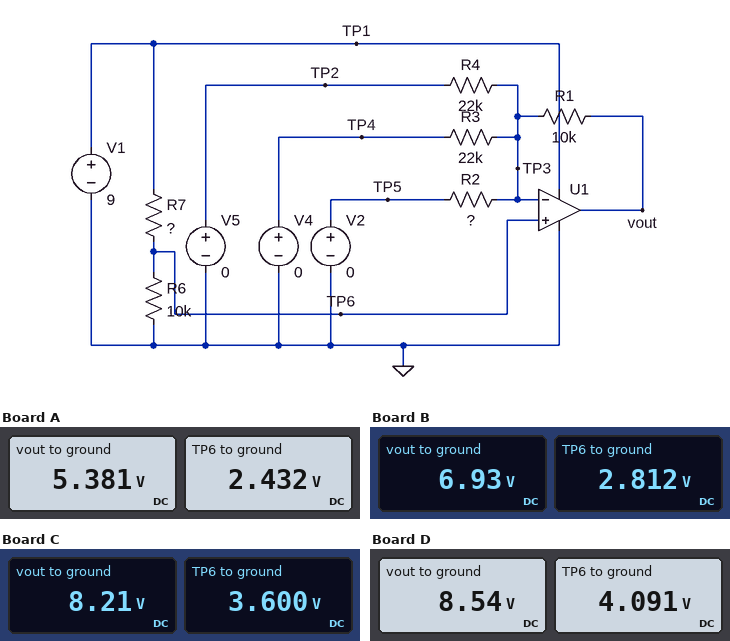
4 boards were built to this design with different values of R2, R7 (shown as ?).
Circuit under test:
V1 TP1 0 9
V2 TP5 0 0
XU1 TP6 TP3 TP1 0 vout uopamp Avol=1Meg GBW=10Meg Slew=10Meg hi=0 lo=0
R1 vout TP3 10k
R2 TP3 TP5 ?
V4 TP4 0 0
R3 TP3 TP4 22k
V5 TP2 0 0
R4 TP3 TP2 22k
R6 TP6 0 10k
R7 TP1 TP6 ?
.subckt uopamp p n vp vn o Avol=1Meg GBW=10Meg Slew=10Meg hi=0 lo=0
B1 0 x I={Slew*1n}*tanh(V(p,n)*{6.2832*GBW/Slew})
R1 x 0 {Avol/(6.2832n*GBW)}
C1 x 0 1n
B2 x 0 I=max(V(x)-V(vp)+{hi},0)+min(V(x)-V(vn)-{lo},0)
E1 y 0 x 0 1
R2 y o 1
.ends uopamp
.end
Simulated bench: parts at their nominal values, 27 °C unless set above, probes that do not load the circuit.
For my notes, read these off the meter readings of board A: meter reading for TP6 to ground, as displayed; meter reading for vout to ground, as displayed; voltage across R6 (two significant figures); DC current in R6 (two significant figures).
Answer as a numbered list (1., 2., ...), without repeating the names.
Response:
1. 2.432 V
2. 5.381 V
3. 2.4 V
4. 240 µA
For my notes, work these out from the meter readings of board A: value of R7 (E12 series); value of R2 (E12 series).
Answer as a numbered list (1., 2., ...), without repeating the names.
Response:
1. 27 kΩ
2. 33 kΩ
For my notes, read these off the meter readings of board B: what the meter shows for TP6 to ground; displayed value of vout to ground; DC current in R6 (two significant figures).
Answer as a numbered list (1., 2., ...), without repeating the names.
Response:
1. 2.812 V
2. 6.93 V
3. 280 µA
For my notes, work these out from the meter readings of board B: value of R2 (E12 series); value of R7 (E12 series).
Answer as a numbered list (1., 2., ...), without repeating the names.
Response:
1. 18 kΩ
2. 22 kΩ
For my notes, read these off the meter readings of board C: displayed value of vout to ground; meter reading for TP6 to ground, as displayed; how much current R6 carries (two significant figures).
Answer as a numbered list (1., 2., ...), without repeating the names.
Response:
1. 8.21 V
2. 3.600 V
3. 360 µA
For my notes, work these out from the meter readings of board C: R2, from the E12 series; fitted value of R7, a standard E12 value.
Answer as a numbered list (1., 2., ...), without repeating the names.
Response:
1. 27 kΩ
2. 15 kΩ
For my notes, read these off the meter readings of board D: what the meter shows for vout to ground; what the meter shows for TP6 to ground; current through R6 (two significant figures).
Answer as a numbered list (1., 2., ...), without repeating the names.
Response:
1. 8.54 V
2. 4.091 V
3. 410 µA
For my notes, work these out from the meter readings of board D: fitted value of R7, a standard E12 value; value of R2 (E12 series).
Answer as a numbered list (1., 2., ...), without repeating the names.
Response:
1. 12 kΩ
2. 56 kΩ
